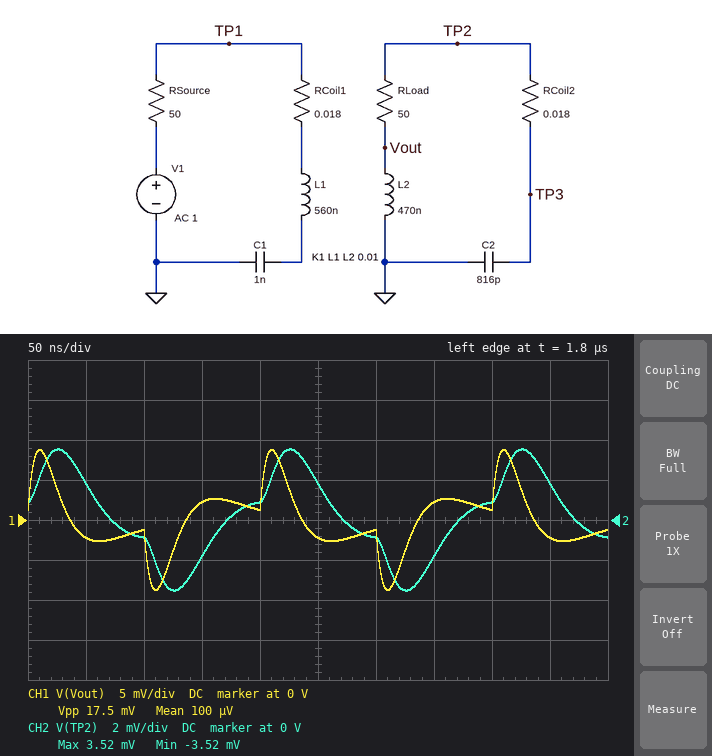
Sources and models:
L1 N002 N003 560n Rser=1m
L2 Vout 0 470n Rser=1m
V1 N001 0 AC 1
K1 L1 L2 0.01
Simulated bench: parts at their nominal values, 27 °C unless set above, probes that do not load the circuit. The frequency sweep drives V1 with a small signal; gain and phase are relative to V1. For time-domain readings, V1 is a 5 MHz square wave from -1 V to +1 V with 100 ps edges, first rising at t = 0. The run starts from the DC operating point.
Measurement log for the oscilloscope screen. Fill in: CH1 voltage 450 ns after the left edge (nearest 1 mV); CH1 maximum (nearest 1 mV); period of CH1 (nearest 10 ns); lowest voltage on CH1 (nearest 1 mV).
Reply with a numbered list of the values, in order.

1. -2 mV
2. 9 mV
3. 200 ns
4. -9 mV
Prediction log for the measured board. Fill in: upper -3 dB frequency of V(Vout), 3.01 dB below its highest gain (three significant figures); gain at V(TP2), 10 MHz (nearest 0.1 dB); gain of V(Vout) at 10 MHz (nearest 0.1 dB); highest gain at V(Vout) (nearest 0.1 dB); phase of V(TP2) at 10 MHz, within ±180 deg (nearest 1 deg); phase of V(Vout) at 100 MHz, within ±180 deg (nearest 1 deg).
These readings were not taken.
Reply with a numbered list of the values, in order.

1. 28.9 MHz
2. -52.8 dB
3. -44.0 dB
4. -43.6 dB
5. -32 deg
6. -74 deg
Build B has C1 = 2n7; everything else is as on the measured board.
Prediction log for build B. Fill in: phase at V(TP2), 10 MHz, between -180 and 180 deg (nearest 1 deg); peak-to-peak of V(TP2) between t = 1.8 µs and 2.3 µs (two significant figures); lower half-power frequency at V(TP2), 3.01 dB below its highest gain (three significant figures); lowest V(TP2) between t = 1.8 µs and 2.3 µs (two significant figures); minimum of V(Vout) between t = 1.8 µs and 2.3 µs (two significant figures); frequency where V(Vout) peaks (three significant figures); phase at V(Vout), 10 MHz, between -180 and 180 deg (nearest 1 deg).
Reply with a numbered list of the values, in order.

1. -42 deg
2. 6.8 mV
3. 3.07 MHz
4. -3.4 mV
5. -8.9 mV
6. 13.2 MHz
7. 27 deg
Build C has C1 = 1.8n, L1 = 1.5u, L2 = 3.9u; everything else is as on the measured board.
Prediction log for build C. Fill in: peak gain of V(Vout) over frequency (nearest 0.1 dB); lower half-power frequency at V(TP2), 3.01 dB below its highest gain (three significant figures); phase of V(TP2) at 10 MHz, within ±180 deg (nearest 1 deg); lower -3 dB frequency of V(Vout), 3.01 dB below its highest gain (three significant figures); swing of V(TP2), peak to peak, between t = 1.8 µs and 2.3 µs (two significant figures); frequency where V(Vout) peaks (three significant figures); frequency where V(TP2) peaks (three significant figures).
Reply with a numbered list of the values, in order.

1. -36.6 dB
2. 2.10 MHz
3. -137 deg
4. 2.20 MHz
5. 14 mV
6. 2.98 MHz
7. 2.86 MHz
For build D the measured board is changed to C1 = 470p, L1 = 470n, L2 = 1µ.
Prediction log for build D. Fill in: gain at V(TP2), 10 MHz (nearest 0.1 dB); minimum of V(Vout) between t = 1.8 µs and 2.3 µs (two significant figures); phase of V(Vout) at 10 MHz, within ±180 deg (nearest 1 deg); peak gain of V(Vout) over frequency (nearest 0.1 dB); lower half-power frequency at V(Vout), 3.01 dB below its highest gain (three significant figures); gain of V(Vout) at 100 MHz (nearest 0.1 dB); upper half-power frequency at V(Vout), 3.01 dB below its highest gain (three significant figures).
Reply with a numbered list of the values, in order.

1. -51.9 dB
2. -7.7 mV
3. 33 deg
4. -43.1 dB
5. 6.11 MHz
6. -58.7 dB
7. 21.9 MHz
